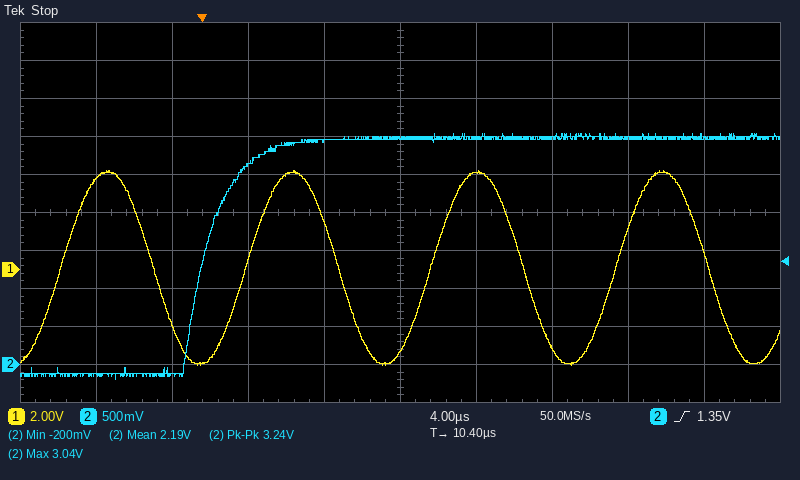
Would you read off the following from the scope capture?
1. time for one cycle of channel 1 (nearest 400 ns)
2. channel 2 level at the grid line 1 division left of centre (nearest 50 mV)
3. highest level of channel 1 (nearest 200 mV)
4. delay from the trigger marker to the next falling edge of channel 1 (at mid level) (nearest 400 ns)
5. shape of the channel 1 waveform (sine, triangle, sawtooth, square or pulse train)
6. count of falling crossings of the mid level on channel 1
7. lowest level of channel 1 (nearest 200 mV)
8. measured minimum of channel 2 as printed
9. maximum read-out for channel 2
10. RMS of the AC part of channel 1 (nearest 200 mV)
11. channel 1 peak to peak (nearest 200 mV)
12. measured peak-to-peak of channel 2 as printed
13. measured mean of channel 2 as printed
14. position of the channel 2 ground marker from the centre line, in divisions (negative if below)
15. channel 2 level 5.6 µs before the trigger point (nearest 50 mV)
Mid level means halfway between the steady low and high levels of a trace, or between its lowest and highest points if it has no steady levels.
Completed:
9.6 µs
2.95 V
5.2 V
7.2 µs
sine
4
-5.0 V
-200 mV
3.04 V
3.6 V
10.2 V
3.24 V
2.19 V
-4.0 div
-150 mV
